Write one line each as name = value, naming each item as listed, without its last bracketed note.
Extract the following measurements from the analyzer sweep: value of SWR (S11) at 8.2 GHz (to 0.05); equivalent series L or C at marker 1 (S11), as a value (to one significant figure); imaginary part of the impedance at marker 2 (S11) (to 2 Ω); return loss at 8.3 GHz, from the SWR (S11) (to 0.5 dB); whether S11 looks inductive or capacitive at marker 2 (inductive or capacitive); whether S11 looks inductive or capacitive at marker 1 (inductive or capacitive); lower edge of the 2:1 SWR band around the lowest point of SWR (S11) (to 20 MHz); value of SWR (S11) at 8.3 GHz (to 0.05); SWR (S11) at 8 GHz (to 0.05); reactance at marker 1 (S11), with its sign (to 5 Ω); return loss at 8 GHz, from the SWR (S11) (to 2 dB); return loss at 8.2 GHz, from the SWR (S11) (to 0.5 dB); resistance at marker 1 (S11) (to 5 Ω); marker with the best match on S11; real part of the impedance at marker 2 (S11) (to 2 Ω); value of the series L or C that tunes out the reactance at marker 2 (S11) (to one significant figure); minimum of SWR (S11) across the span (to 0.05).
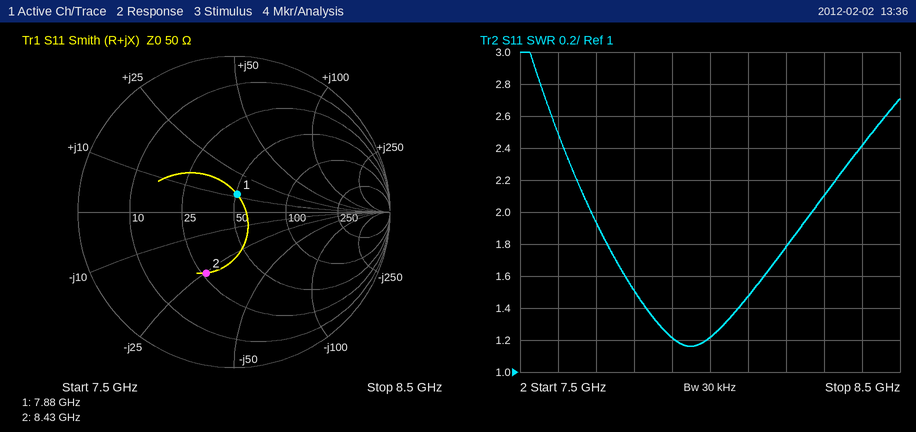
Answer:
value of SWR (S11) at 8.2 GHz = 1.80
equivalent series L or C at marker 1 (S11), as a value = 200 pH
imaginary part of the impedance at marker 2 (S11) = -26 Ω
return loss at 8.3 GHz, from the SWR (S11) = 9.0 dB
whether S11 looks inductive or capacitive at marker 2 = capacitive
whether S11 looks inductive or capacitive at marker 1 = inductive
lower edge of the 2:1 SWR band around the lowest point of SWR (S11) = 7.68 GHz
value of SWR (S11) at 8.3 GHz = 2.10
SWR (S11) at 8 GHz = 1.20
reactance at marker 1 (S11), with its sign = +10 Ω
return loss at 8 GHz, from the SWR (S11) = 20 dB
return loss at 8.2 GHz, from the SWR (S11) = 11.0 dB
resistance at marker 1 (S11) = 50 Ω
marker with the best match on S11 = marker 1
real part of the impedance at marker 2 (S11) = 26 Ω
value of the series L or C that tunes out the reactance at marker 2 (S11) = 500 pH
minimum of SWR (S11) across the span = 1.15
